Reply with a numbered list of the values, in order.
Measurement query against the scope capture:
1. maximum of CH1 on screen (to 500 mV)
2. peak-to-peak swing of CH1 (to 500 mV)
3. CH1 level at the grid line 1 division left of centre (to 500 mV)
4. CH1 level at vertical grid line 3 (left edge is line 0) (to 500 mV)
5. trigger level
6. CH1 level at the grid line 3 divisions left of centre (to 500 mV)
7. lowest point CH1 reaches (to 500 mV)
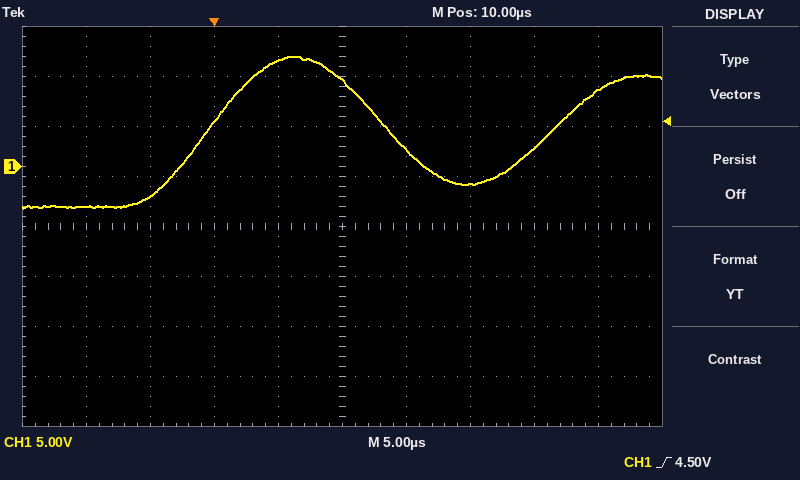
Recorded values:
1. 11.0 V
2. 15.0 V
3. 10.5 V
4. 4.5 V
5. 4.50 V
6. -3.0 V
7. -4.0 V
